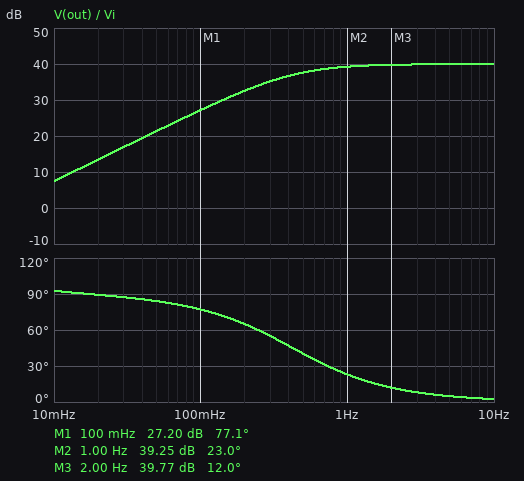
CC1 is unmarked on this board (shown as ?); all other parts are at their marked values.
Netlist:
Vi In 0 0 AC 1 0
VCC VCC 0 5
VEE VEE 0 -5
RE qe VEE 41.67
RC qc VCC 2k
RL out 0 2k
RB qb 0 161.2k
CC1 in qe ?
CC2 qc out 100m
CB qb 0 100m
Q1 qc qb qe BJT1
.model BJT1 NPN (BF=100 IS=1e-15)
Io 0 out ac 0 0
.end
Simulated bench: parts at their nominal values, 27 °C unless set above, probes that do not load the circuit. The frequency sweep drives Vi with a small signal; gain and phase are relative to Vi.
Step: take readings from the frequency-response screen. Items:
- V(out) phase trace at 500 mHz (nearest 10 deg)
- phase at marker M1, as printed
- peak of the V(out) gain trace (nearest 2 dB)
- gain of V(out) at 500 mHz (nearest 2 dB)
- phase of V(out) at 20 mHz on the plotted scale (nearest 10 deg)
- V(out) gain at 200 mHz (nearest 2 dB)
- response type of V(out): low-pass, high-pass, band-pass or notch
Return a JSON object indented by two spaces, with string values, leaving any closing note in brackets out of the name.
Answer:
{
  "V(out) phase trace at 500 mHz": "40 deg",
  "phase at marker M1, as printed": "77.1 deg",
  "peak of the V(out) gain trace": "40 dB",
  "gain of V(out) at 500 mHz": "38 dB",
  "phase of V(out) at 20 mHz on the plotted scale": "90 deg",
  "V(out) gain at 200 mHz": "32 dB",
  "response type of V(out): low-pass, high-pass, band-pass or notch": "high-pass"
}
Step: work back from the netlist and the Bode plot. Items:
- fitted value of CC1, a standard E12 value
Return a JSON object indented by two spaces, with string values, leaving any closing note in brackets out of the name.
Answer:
{
  "fitted value of CC1, a standard E12 value": "47 mF"
}
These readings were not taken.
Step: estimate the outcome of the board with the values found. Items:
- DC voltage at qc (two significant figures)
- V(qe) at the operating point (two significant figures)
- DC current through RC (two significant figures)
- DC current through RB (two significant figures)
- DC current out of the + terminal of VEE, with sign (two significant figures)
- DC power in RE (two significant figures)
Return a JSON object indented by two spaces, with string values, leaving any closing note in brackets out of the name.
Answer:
{
  "DC voltage at qc": "-150 mV",
  "V(qe) at the operating point": "-4.9 V",
  "DC current through RC": "2.6 mA",
  "DC current through RB": "26 µA",
  "DC current out of the + terminal of VEE, with sign": "-2.6 mA",
  "DC power in RE": "280 µW"
}
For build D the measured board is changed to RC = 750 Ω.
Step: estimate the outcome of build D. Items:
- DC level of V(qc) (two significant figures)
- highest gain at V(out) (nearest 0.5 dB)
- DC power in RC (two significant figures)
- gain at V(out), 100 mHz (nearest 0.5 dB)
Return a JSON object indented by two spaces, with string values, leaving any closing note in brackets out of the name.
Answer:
{
  "DC level of V(qc)": "3.1 V",
  "highest gain at V(out)": "34.5 dB",
  "DC power in RC": "5.0 mW",
  "gain at V(out), 100 mHz": "22.0 dB"
}
